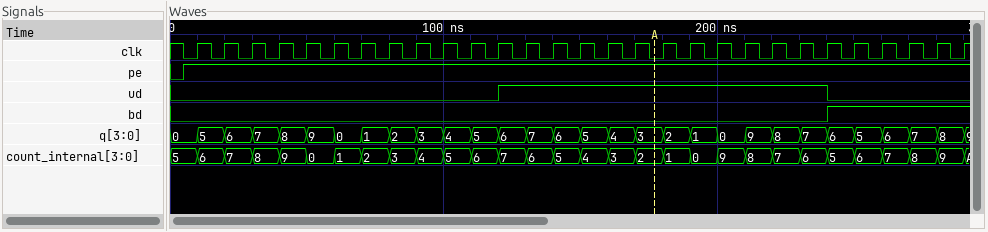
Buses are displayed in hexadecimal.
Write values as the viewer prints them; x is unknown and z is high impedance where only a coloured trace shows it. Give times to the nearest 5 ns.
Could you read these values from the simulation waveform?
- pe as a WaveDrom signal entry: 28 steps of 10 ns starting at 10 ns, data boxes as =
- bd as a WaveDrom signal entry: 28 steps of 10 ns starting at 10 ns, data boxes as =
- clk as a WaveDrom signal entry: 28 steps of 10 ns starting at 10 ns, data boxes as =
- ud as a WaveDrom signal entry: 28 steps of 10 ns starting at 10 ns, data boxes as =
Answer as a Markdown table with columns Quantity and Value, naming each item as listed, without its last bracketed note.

| Quantity | Value |
|---|---|
| pe as a WaveDrom signal entry: 28 steps of 10 ns starting at 10 ns, data boxes as = | {name: 'pe', wave: '1...........................'} |
| bd as a WaveDrom signal entry: 28 steps of 10 ns starting at 10 ns, data boxes as = | {name: 'bd', wave: '0......................1....'} |
| clk as a WaveDrom signal entry: 28 steps of 10 ns starting at 10 ns, data boxes as = | {name: 'clk', wave: 'p...........................'} |
| ud as a WaveDrom signal entry: 28 steps of 10 ns starting at 10 ns, data boxes as = | {name: 'ud', wave: '0..........1...........0....'} |
